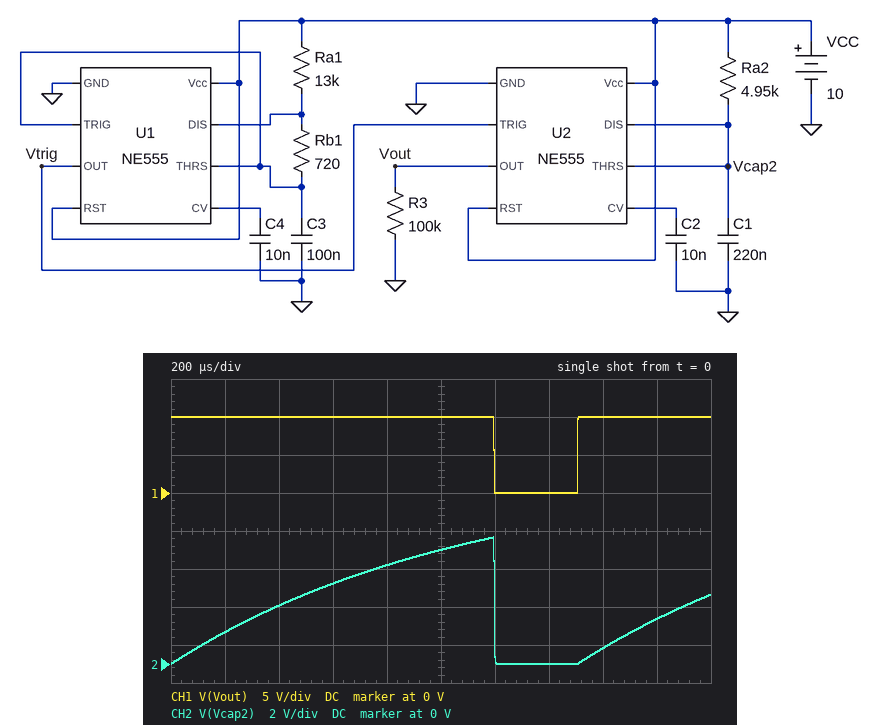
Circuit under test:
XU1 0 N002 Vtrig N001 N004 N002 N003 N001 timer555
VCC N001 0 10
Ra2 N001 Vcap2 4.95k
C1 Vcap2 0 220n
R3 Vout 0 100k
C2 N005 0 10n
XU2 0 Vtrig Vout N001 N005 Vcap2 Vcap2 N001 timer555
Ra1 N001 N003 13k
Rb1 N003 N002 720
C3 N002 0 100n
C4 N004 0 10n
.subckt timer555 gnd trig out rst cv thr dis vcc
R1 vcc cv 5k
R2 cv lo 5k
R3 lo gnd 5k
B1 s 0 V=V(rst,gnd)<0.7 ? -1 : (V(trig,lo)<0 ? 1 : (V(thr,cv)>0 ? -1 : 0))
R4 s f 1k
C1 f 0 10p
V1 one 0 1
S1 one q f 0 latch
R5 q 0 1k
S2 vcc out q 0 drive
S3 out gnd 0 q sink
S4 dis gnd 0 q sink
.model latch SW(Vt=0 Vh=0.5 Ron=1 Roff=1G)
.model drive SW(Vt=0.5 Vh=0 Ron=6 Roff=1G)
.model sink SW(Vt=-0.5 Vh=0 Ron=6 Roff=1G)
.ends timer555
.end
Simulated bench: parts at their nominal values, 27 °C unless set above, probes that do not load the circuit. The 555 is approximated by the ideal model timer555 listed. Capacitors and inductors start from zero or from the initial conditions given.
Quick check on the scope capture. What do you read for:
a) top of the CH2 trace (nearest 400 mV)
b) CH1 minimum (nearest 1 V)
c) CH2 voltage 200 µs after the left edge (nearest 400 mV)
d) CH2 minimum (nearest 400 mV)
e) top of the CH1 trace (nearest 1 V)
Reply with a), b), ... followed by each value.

a) 6.8 V
b) 0 V
c) 1.6 V
d) 0 V
e) 10 V
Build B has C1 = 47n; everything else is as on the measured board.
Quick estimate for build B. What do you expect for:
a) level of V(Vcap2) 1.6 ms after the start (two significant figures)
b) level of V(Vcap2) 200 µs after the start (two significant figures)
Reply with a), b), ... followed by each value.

a) 3.3 V
b) 5.8 V
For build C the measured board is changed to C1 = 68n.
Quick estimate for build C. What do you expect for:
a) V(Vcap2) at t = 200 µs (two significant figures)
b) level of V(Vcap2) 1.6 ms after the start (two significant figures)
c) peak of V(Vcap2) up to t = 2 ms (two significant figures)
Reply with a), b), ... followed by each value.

a) 4.5 V
b) 2.4 V
c) 6.7 V
